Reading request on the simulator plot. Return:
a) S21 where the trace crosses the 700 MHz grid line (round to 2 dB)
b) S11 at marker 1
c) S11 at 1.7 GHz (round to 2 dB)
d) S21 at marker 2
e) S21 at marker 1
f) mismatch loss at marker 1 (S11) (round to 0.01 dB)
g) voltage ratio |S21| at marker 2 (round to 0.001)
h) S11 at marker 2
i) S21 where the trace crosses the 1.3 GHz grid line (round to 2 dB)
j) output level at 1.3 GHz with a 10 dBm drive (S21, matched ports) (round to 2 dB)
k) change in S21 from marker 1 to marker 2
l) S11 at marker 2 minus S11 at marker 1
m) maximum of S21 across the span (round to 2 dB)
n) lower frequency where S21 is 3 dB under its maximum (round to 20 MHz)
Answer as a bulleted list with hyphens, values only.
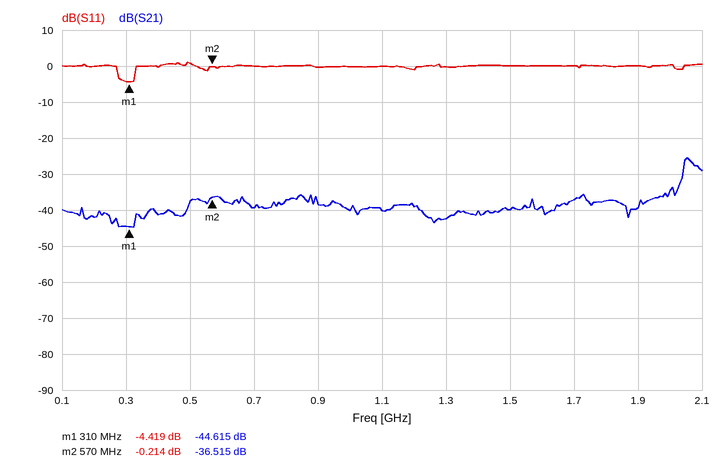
- -40 dB
- -4.419 dB
- 0 dB
- -36.515 dB
- -44.615 dB
- 1.95 dB
- 0.015
- -0.214 dB
- -42 dB
- -32 dBm
- 8.100 dB
- 4.205 dB
- -26 dB
- 2.04 GHz
